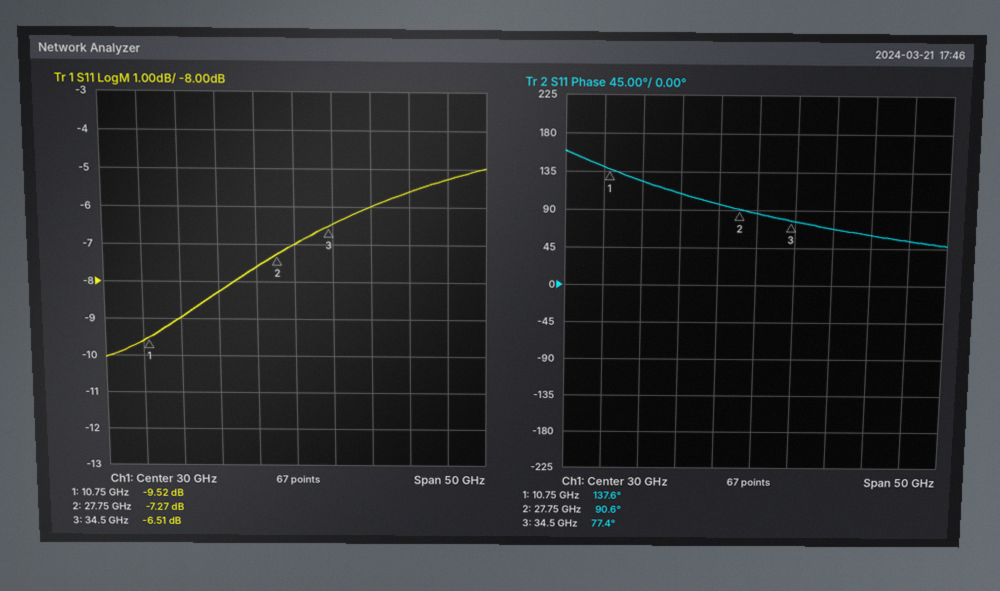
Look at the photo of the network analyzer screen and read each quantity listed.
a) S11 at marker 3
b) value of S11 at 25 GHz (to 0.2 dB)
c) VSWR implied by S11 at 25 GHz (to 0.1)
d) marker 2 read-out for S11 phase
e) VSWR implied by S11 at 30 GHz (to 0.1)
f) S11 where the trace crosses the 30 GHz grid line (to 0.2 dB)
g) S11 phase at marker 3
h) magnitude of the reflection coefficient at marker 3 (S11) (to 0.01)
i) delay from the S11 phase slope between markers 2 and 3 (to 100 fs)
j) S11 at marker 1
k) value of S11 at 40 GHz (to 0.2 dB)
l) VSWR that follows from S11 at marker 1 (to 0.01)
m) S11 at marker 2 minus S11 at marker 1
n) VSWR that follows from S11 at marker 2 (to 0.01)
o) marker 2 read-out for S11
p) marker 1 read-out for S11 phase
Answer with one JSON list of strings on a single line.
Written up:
["-6.51 dB", "-7.6 dB", "2.4", "90.6°", "2.6", "-7.0 dB", "77.4°", "0.47", "5.4 ps", "-9.52 dB", "-6.0 dB", "2.00", "2.25 dB", "2.53", "-7.27 dB", "137.6°"]
